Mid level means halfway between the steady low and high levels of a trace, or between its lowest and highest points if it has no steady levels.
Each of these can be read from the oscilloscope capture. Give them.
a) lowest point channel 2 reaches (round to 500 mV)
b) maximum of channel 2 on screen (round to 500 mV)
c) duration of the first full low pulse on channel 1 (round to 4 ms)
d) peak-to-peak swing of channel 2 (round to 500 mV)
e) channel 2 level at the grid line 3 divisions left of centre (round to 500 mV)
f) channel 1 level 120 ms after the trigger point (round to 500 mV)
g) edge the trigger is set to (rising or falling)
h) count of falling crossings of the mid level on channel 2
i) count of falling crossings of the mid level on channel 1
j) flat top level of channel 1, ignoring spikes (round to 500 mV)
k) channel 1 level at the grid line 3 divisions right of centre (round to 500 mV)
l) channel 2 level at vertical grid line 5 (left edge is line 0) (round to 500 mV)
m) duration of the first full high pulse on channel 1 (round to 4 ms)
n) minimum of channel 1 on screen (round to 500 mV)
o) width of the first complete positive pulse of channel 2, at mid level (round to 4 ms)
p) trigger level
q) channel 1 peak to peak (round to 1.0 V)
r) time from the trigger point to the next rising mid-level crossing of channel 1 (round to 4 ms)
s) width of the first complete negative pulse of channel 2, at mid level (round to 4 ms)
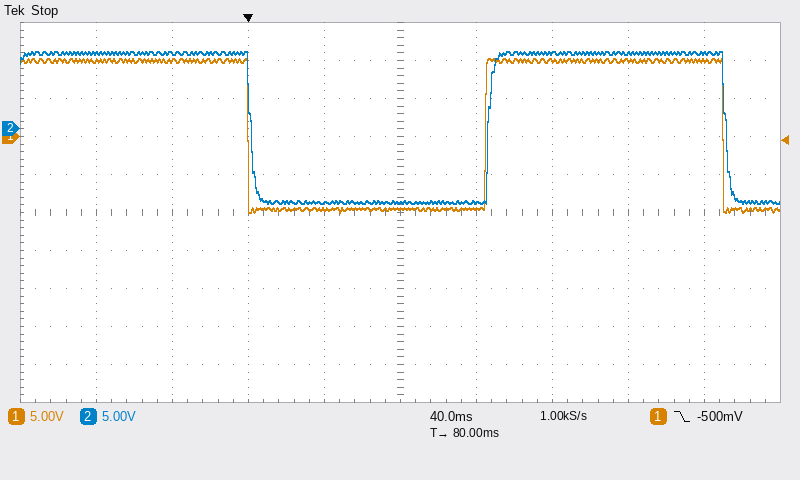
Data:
-10.0 V
10.0 V
124 ms
20.0 V
10.0 V
-9.5 V
falling
2
2
10.0 V
10.0 V
-9.5 V
124 ms
-10.0 V
124 ms
-500 mV
20.0 V
124 ms
124 ms
